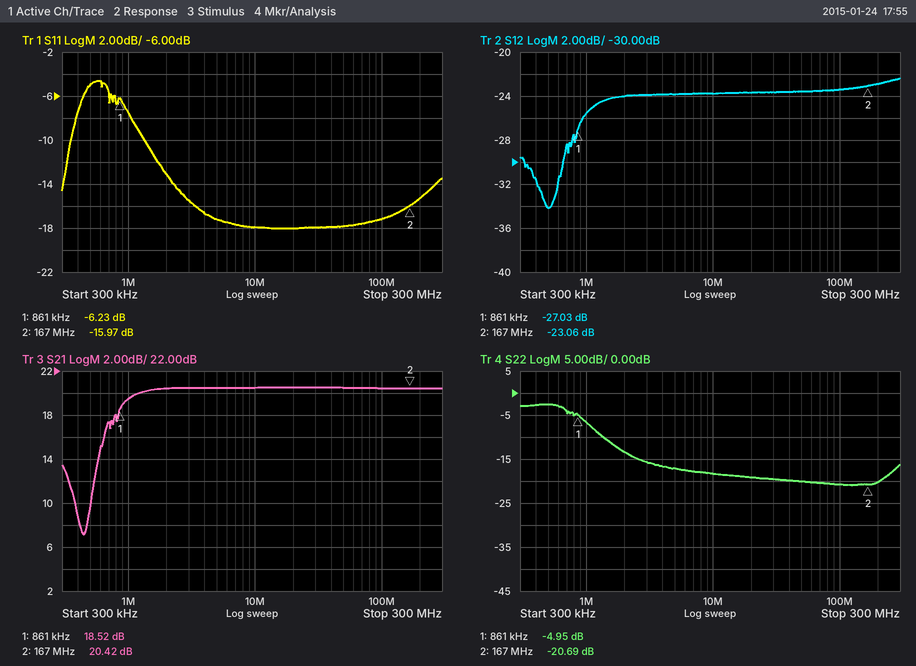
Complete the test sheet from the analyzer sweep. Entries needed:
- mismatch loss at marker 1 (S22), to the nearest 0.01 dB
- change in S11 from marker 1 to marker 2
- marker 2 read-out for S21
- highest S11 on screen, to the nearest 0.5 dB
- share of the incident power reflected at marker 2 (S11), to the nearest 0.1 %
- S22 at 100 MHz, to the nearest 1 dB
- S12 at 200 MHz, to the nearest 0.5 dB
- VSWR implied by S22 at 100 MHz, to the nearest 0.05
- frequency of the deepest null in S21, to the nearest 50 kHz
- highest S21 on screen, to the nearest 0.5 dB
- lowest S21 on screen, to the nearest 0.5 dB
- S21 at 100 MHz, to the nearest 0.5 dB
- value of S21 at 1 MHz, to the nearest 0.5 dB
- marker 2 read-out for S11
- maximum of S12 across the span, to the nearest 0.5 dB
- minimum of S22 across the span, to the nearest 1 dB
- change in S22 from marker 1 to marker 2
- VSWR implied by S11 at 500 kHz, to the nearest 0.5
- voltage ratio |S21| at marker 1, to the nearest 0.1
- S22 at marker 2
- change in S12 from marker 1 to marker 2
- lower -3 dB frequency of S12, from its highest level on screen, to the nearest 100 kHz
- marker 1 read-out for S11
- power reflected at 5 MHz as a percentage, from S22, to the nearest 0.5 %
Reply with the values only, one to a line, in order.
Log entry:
1.67 dB
-9.74 dB
20.42 dB
-4.5 dB
2.5 %
-21 dB
-23.0 dB
1.20
450 kHz
20.5 dB
7.0 dB
20.5 dB
19.5 dB
-15.97 dB
-22.5 dB
-21 dB
-15.74 dB
3.5
8.4
-20.69 dB
3.97 dB
1.0 MHz
-6.23 dB
2.0 %
